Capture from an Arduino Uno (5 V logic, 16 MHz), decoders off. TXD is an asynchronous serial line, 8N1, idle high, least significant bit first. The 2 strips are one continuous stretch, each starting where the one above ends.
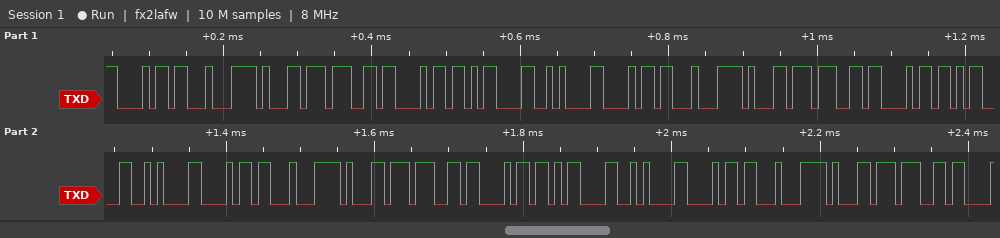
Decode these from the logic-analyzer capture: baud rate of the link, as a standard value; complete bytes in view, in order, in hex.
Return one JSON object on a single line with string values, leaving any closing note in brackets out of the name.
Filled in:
{"baud rate of the link, as a standard value": "115200 baud", "complete bytes in view, in order, in hex": "68 C4 B1 67 68 0D 0A 68 C4 B1 67 68 0D 0A 68 C4 B1 67 68 0D 0A 68 C4 B1 67"}
